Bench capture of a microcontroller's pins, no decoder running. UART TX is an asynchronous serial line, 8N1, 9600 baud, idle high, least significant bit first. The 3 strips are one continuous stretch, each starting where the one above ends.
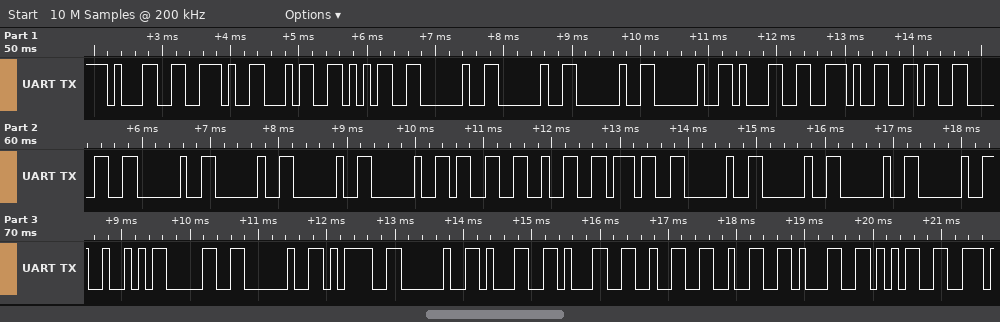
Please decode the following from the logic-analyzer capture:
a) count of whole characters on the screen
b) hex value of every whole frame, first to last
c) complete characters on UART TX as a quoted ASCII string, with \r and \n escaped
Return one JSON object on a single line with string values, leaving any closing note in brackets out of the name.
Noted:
{"count of whole characters on the screen": "34", "hex value of every whole frame, first to last": "31 2E 34 35 20 20 20 20 31 2E 36 30 20 20 20 20 33 32 37 20 20 20 20 52 30 20 3D 20 31 31 32 32 31 35", "complete characters on UART TX as a quoted ASCII string, with \\r and \\n escaped": "\"1.45    1.60    327    R0 = 112215\""}
